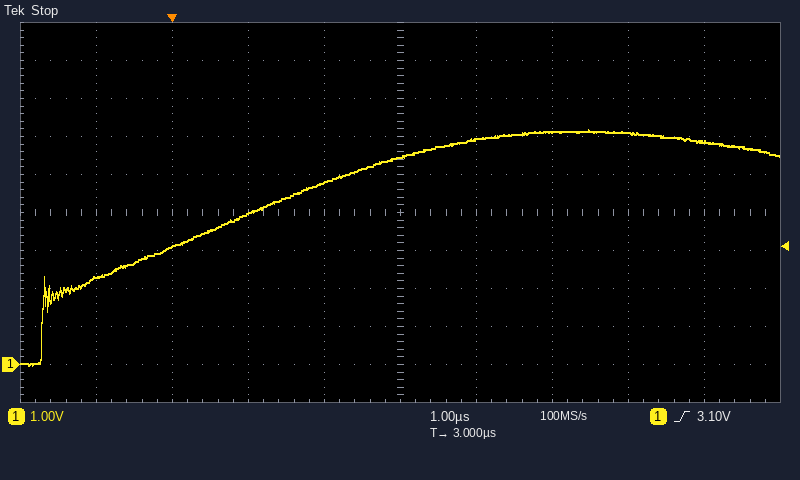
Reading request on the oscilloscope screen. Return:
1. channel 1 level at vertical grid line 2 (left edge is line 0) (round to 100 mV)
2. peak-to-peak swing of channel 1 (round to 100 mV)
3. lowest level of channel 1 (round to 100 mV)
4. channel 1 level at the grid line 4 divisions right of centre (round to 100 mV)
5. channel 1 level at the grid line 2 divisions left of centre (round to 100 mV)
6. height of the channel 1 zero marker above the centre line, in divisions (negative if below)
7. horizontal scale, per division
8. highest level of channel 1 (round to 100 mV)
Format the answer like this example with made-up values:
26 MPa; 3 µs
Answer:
3.1 V; 6.2 V; 0.0 V; 5.9 V; 4.0 V; -4.0 div; 1 µs; 6.2 V
